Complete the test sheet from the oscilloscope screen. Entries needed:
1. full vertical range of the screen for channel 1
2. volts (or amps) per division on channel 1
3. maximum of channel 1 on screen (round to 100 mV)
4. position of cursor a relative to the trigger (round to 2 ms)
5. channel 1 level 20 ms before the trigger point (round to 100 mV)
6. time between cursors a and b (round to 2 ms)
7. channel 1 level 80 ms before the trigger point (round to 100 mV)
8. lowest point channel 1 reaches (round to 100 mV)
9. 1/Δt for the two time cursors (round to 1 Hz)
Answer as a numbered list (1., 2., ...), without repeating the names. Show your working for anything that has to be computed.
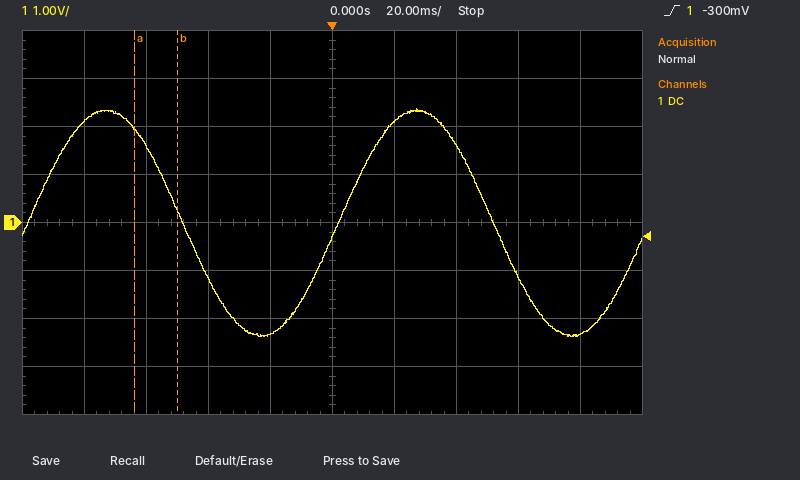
1. 8 V
2. 1 V
3. 2.4 V
4. -64 ms
5. -2.3 V
6. 14 ms
7. 2.1 V
8. -2.4 V
9. 1 / 14 ms ≈ 71 Hz
